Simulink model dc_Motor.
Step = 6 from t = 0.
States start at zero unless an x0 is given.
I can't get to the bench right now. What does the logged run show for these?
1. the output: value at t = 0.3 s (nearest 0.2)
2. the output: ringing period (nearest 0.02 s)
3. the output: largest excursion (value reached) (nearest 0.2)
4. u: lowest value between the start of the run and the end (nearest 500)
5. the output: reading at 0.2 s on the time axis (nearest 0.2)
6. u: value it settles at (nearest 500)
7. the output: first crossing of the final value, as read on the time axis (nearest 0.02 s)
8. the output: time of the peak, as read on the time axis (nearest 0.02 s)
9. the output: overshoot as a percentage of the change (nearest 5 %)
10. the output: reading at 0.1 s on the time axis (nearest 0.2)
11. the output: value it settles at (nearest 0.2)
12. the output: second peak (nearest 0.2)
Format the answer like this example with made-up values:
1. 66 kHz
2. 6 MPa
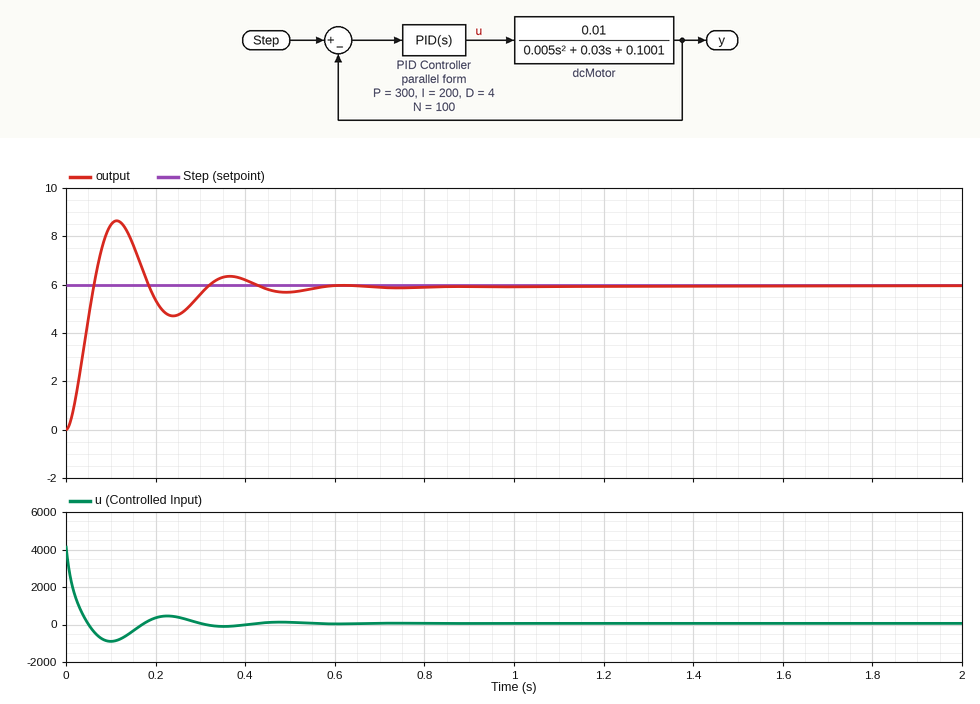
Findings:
1. 5.6
2. 0.26 s
3. 8.6
4. -1000
5. 5.4
6. 0
7. 0.06 s
8. 0.12 s
9. 45 %
10. 8.4
11. 6.0
12. 6.4
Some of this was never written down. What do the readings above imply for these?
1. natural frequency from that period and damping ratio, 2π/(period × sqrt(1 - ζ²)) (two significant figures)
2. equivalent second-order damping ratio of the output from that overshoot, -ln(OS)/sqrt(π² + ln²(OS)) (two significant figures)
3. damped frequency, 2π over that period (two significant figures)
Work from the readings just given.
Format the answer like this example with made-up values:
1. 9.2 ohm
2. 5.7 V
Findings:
1. 25 rad/s
2. 0.25
3. 24 rad/s
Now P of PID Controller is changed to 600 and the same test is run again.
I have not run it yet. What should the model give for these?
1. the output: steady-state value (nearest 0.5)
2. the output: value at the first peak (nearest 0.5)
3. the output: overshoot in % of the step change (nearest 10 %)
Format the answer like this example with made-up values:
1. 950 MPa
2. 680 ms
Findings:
1. 6.0
2. 9.5
3. 60 %
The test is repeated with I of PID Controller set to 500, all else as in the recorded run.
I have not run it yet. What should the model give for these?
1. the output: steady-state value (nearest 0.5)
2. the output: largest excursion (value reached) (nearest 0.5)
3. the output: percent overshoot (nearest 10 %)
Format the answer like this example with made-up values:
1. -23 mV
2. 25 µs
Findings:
1. 6.0
2. 9.0
3. 50 %
